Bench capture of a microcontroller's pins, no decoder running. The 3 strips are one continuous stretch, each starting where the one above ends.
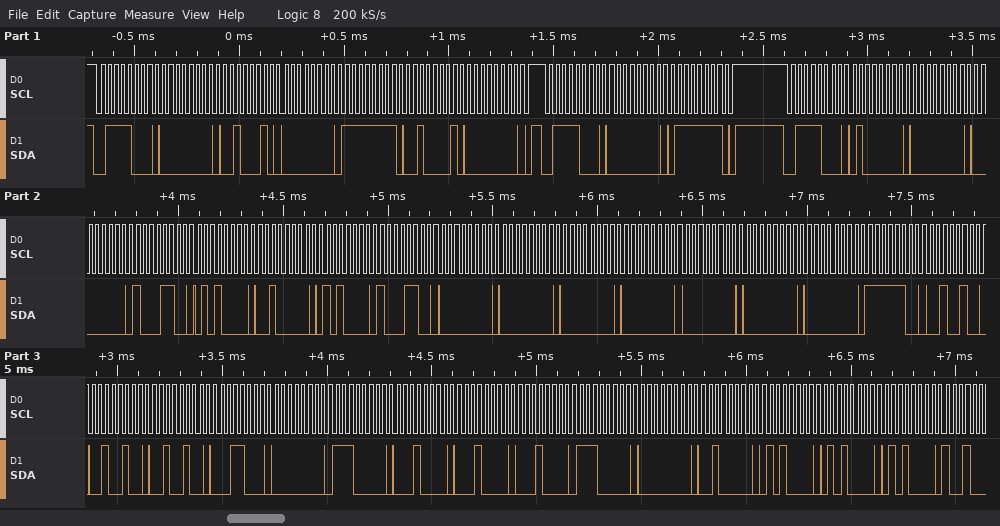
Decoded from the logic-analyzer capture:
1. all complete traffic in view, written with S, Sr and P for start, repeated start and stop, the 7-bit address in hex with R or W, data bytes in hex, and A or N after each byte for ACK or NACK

S 3CW A 00 A 22 A 00 A FF A 21 A 00 A P S 3CW A 00 A 7F A P S 3CW A 40 A 00 A 00 A 8C A 50 A 20 A 50 A 8C A 00 A 00 A 00 A 00 A 00 A 00 A 00 A FC A 24 A 24 A 24 A 18 A 00 A E0 A 10 A 10 A 10 A E0 A 00 A 20 A 50 A 50 A 50 A
